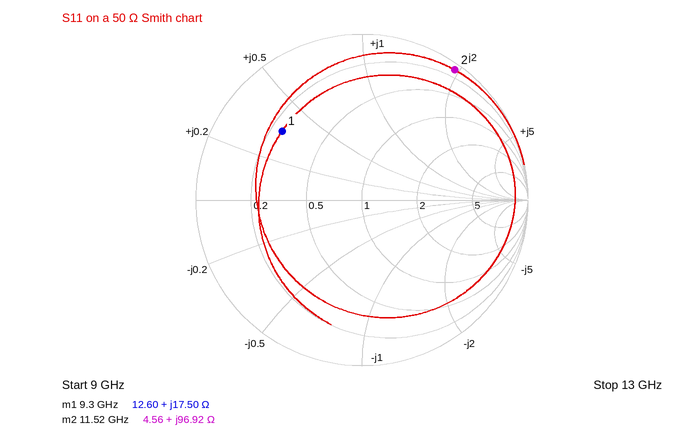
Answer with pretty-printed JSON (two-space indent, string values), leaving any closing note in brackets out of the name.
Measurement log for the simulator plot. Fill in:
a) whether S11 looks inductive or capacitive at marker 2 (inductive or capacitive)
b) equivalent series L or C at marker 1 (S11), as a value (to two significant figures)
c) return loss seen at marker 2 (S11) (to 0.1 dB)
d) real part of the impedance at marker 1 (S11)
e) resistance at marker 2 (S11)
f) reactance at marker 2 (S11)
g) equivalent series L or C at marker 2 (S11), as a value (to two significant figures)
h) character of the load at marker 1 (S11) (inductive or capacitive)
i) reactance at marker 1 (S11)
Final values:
{
  "whether S11 looks inductive or capacitive at marker 2": "inductive",
  "equivalent series L or C at marker 1 (S11), as a value": "300 pH",
  "return loss seen at marker 2 (S11)": "0.3 dB",
  "real part of the impedance at marker 1": "12.60 Ω",
  "resistance at marker 2": "4.56 Ω",
  "reactance at marker 2": "+96.92 Ω",
  "equivalent series L or C at marker 2 (S11), as a value": "1.3 nH",
  "character of the load at marker 1 (S11)": "inductive",
  "reactance at marker 1": "+17.50 Ω"
}
